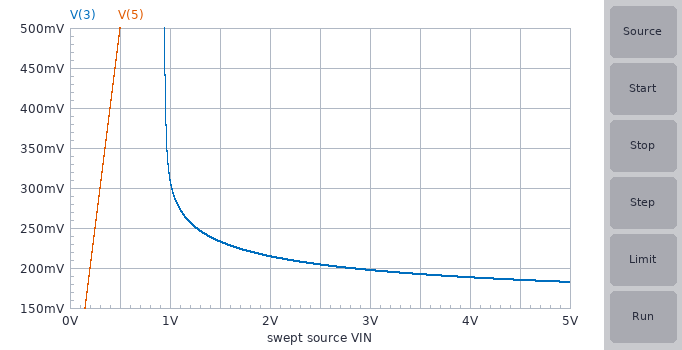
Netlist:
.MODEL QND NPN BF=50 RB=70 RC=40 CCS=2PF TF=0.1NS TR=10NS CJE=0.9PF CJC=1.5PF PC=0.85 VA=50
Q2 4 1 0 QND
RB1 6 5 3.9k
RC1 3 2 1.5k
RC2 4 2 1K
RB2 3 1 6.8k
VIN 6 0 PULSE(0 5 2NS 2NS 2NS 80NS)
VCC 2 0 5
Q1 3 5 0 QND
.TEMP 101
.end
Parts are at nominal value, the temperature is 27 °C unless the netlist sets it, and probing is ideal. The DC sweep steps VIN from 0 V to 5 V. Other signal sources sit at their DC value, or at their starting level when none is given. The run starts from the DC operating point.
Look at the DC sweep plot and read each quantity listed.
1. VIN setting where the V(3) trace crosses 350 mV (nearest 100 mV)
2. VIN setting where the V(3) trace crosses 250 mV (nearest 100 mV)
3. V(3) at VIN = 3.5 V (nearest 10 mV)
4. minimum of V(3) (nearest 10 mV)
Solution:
1.0 V
1.3 V
190 mV
180 mV
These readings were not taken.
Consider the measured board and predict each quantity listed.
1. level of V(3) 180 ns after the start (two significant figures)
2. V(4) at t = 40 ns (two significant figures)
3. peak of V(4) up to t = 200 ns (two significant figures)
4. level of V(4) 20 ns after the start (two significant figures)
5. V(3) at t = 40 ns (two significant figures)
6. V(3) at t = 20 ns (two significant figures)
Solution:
4.2 V
2.1 V
5.0 V
380 mV
190 mV
200 mV
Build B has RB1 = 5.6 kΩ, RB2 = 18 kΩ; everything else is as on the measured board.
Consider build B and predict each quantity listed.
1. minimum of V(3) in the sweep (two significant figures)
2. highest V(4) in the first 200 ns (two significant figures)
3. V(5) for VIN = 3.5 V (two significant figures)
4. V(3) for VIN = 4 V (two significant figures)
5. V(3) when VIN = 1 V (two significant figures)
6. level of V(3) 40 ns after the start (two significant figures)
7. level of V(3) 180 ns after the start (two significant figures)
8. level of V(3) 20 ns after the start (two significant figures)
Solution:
190 mV
4.6 V
750 mV
200 mV
1.0 V
190 mV
4.7 V
210 mV
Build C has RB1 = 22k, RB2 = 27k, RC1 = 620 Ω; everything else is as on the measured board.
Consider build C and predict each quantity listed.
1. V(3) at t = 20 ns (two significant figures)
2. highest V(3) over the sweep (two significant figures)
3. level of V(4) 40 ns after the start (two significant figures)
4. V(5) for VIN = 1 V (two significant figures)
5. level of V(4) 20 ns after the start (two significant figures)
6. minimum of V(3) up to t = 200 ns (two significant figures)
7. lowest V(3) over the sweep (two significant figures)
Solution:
3.5 V
4.9 V
500 mV
660 mV
340 mV
490 mV
460 mV
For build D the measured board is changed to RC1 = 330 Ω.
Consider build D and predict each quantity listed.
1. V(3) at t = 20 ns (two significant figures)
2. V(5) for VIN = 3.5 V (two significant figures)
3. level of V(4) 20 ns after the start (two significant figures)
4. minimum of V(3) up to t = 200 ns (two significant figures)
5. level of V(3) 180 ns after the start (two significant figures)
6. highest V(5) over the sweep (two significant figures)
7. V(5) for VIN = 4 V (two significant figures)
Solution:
640 mV
800 mV
320 mV
630 mV
4.8 V
830 mV
810 mV
